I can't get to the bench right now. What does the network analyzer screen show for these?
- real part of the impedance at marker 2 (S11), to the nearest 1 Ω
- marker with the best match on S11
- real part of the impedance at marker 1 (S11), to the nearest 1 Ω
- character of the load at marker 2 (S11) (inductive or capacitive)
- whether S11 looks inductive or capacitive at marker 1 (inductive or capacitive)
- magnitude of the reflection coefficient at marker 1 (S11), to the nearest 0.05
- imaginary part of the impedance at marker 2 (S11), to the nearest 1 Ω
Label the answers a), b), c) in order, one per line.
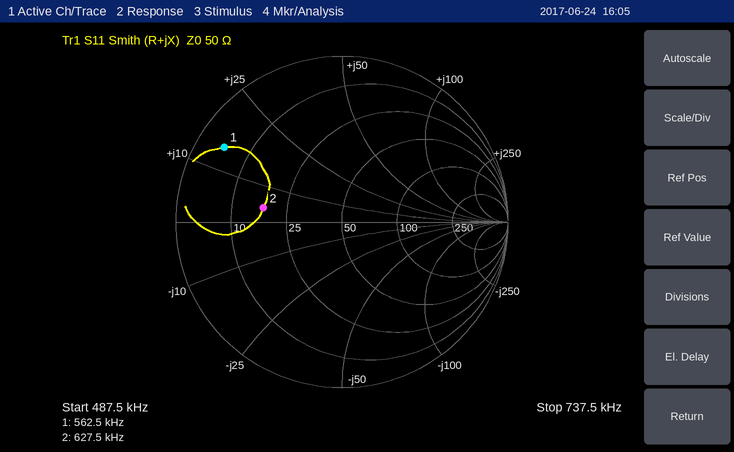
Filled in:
a) 18 Ω
b) marker 2
c) 5 Ω
d) inductive
e) inductive
f) 0.85
g) +4 Ω
